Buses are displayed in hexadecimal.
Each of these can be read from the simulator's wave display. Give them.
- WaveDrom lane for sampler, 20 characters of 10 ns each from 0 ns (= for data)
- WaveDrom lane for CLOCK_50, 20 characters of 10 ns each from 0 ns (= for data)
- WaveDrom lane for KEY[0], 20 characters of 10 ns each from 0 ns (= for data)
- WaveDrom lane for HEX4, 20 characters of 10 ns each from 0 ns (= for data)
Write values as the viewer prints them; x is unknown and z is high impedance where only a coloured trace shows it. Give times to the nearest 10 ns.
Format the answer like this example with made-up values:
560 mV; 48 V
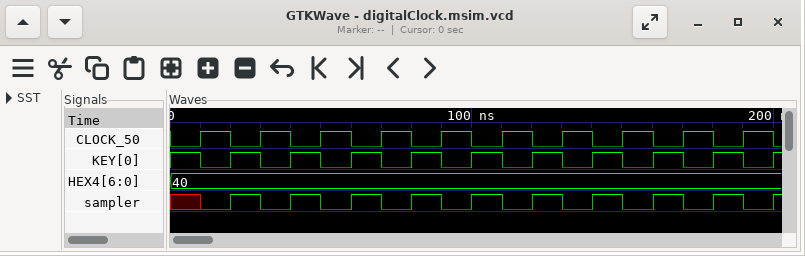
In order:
{name: 'sampler', wave: 'x0101010101010101010'}; {name: 'CLOCK_50', wave: '01010101010101010101'}; {name: 'KEY[0]', wave: '10101010101010101010'}; {name: 'HEX4', wave: '=...................', data: '40'}
